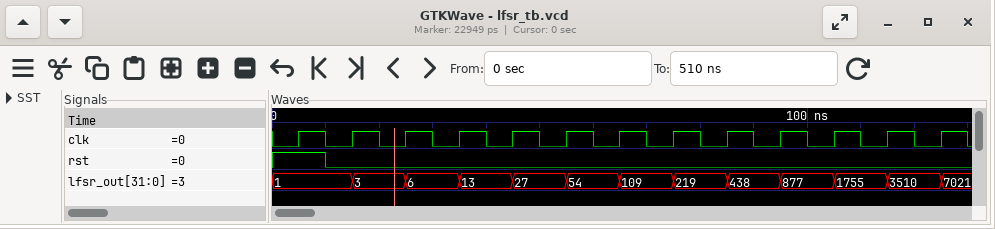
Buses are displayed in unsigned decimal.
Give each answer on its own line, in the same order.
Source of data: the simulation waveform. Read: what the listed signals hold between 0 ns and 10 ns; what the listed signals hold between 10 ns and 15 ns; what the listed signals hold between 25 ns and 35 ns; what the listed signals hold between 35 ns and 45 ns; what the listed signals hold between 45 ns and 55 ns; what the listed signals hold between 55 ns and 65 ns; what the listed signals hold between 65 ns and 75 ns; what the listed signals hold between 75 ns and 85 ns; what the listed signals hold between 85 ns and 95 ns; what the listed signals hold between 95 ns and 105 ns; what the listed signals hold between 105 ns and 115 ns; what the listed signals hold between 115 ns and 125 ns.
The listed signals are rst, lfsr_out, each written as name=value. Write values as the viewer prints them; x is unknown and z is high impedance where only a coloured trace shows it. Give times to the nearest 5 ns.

rst=1, lfsr_out=1
rst=0, lfsr_out=1
rst=0, lfsr_out=6
rst=0, lfsr_out=13
rst=0, lfsr_out=27
rst=0, lfsr_out=54
rst=0, lfsr_out=109
rst=0, lfsr_out=219
rst=0, lfsr_out=438
rst=0, lfsr_out=877
rst=0, lfsr_out=1755
rst=0, lfsr_out=3510
